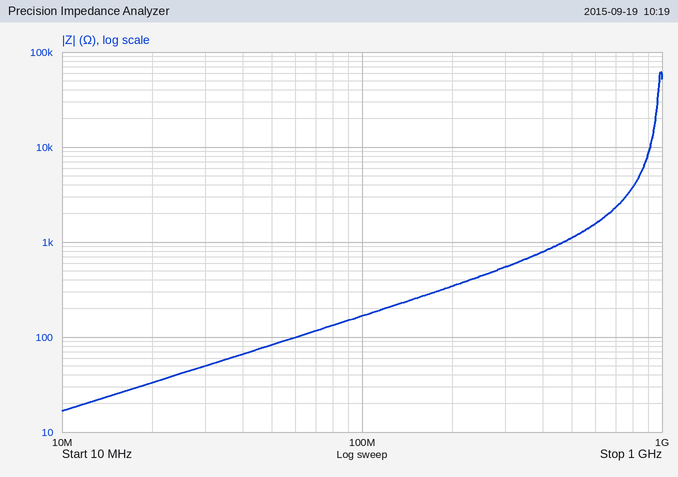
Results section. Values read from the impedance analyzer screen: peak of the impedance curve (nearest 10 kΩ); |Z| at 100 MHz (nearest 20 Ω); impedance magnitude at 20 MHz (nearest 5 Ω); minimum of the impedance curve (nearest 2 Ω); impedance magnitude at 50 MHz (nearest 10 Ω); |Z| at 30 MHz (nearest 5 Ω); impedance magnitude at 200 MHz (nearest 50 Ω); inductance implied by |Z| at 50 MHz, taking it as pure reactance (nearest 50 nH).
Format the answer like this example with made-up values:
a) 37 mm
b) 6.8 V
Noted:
a) 60 kΩ
b) 160 Ω
c) 35 Ω
d) 16 Ω
e) 80 Ω
f) 50 Ω
g) 350 Ω
h) 250 nH
